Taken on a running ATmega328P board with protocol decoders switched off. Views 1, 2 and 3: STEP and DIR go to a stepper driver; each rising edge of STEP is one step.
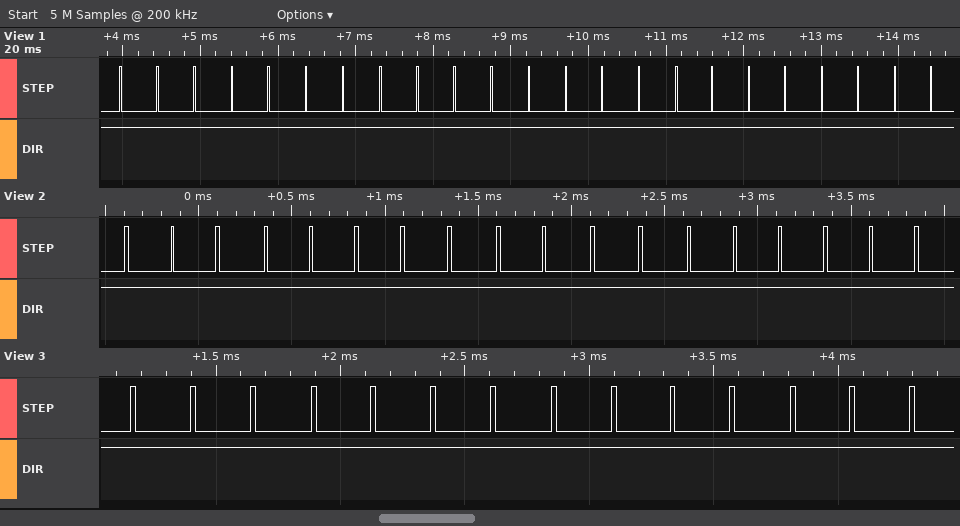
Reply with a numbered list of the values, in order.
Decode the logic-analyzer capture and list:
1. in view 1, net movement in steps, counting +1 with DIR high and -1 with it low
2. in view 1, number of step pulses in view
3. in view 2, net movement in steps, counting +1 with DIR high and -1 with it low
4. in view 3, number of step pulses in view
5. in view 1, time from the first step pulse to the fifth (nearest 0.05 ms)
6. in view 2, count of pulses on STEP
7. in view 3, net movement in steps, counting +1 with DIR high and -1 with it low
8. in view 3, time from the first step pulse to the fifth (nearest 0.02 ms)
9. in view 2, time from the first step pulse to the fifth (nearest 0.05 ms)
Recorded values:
1. +23
2. 23
3. +18
4. 14
5. 1.90 ms
6. 18
7. +14
8. 0.96 ms
9. 1.00 ms
